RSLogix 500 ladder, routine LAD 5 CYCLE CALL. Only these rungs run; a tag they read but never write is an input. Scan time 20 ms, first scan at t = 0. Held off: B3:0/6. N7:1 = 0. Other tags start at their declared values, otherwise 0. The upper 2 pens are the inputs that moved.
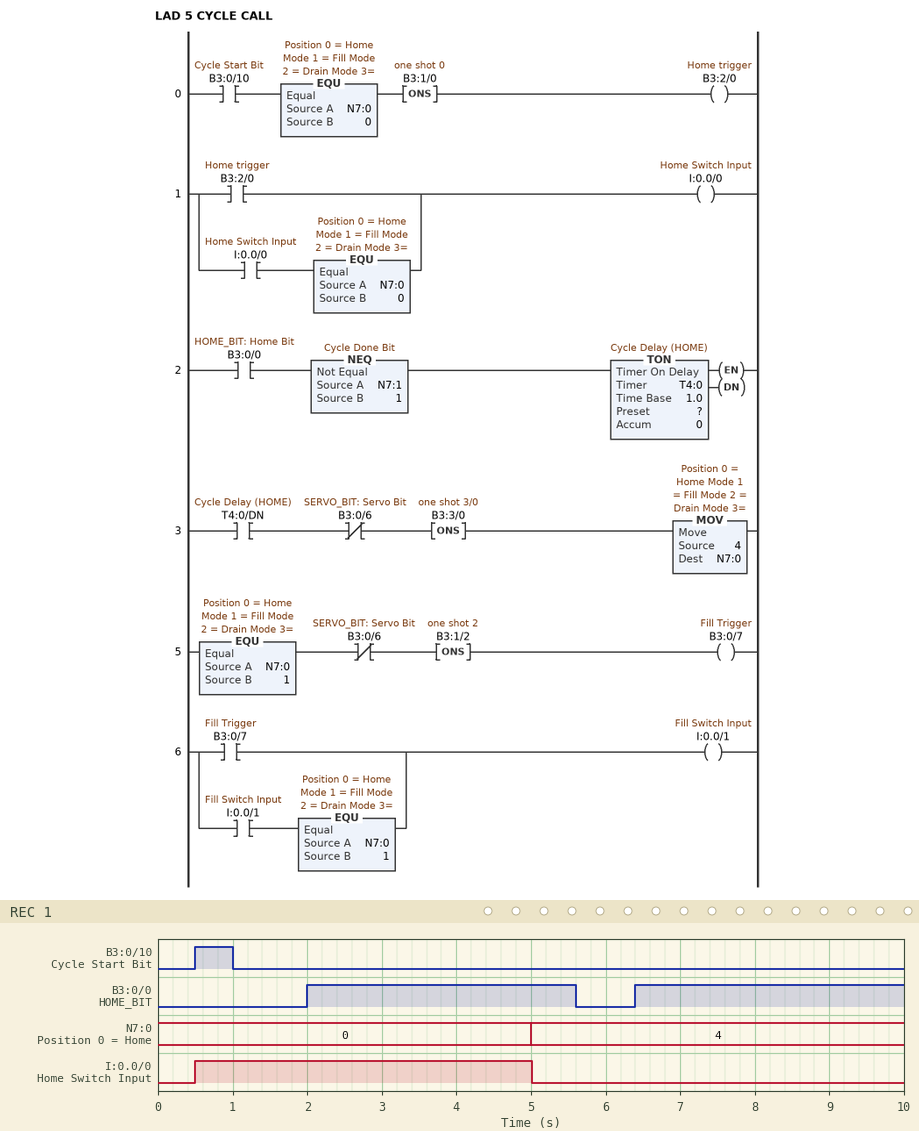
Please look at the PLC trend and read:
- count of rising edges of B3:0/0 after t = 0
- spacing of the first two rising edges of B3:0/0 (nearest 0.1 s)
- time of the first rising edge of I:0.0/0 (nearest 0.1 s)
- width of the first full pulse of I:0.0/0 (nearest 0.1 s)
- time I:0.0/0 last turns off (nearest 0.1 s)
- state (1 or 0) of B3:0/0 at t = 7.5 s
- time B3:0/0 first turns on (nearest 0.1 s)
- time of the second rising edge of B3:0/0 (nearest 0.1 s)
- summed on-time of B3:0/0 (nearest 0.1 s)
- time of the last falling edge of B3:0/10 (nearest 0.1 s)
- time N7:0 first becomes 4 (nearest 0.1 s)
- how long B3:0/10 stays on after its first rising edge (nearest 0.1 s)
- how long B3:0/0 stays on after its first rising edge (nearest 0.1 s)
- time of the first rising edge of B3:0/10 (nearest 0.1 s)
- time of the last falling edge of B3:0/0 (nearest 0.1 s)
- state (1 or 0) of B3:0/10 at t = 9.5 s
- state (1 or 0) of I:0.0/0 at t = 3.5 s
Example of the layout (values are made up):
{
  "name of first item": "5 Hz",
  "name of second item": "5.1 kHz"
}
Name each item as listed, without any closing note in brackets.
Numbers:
{
  "count of rising edges of B3:0/0 after t = 0": "2",
  "spacing of the first two rising edges of B3:0/0": "4.4 s",
  "time of the first rising edge of I:0.0/0": "0.5 s",
  "width of the first full pulse of I:0.0/0": "4.5 s",
  "time I:0.0/0 last turns off": "5.0 s",
  "state (1 or 0) of B3:0/0 at t = 7.5 s": "1",
  "time B3:0/0 first turns on": "2.0 s",
  "time of the second rising edge of B3:0/0": "6.4 s",
  "summed on-time of B3:0/0": "7.2 s",
  "time of the last falling edge of B3:0/10": "1.0 s",
  "time N7:0 first becomes 4": "5.0 s",
  "how long B3:0/10 stays on after its first rising edge": "0.5 s",
  "how long B3:0/0 stays on after its first rising edge": "3.6 s",
  "time of the first rising edge of B3:0/10": "0.5 s",
  "time of the last falling edge of B3:0/0": "5.6 s",
  "state (1 or 0) of B3:0/10 at t = 9.5 s": "0",
  "state (1 or 0) of I:0.0/0 at t = 3.5 s": "1"
}
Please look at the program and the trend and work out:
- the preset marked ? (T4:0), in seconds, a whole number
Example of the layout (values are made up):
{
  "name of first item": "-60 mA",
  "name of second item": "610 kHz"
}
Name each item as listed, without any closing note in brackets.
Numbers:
{
  "the preset marked ? (T4:0), in seconds, a whole number": "3 s"
}
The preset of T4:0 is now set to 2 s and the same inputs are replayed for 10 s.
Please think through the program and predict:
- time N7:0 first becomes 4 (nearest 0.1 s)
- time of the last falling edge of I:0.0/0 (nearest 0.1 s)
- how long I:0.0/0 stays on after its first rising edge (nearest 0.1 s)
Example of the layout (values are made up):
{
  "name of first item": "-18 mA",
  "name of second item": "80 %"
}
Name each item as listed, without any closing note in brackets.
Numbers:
{
  "time N7:0 first becomes 4": "4.0 s",
  "time of the last falling edge of I:0.0/0": "4.0 s",
  "how long I:0.0/0 stays on after its first rising edge": "3.5 s"
}
